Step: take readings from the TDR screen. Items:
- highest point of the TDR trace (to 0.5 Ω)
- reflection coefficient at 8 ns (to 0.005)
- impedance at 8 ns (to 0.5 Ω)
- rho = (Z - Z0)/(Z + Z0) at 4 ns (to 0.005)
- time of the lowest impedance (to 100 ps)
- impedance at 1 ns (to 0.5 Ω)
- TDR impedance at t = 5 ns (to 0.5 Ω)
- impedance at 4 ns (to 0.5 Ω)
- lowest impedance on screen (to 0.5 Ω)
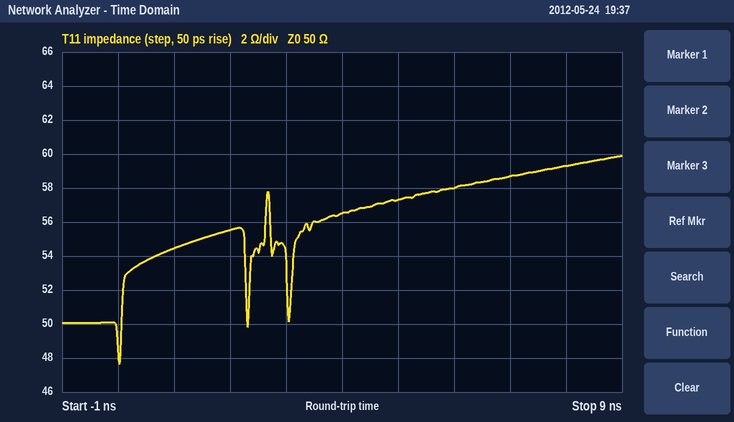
60.0 Ω
+0.085
59.5 Ω
+0.060
0.0 ns
54.5 Ω
57.5 Ω
56.5 Ω
47.5 Ω
